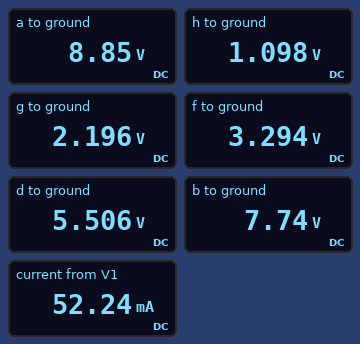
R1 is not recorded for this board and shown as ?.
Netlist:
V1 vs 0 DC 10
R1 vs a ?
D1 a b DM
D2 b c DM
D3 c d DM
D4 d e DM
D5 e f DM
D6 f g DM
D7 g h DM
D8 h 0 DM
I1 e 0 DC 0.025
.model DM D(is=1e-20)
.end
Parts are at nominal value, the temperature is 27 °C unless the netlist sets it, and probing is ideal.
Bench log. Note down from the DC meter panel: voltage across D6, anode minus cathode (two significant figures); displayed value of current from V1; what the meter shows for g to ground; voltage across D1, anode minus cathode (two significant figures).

1.1 V
52.24 mA
2.196 V
1.1 V
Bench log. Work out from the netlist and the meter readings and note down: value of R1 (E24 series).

22 Ω
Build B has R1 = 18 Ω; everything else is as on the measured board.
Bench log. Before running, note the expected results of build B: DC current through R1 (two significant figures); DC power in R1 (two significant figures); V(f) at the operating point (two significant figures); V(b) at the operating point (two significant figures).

61 mA
68 mW
3.3 V
7.8 V
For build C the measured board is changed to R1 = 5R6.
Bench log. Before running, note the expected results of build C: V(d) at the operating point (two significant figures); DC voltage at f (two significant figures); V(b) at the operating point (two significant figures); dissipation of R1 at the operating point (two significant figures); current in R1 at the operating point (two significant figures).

5.7 V
3.4 V
8.0 V
140 mW
160 mA
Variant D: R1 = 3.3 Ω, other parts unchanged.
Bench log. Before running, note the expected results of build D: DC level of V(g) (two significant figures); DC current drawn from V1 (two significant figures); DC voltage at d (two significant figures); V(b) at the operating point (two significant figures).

2.3 V
240 mA
5.8 V
8.1 V
